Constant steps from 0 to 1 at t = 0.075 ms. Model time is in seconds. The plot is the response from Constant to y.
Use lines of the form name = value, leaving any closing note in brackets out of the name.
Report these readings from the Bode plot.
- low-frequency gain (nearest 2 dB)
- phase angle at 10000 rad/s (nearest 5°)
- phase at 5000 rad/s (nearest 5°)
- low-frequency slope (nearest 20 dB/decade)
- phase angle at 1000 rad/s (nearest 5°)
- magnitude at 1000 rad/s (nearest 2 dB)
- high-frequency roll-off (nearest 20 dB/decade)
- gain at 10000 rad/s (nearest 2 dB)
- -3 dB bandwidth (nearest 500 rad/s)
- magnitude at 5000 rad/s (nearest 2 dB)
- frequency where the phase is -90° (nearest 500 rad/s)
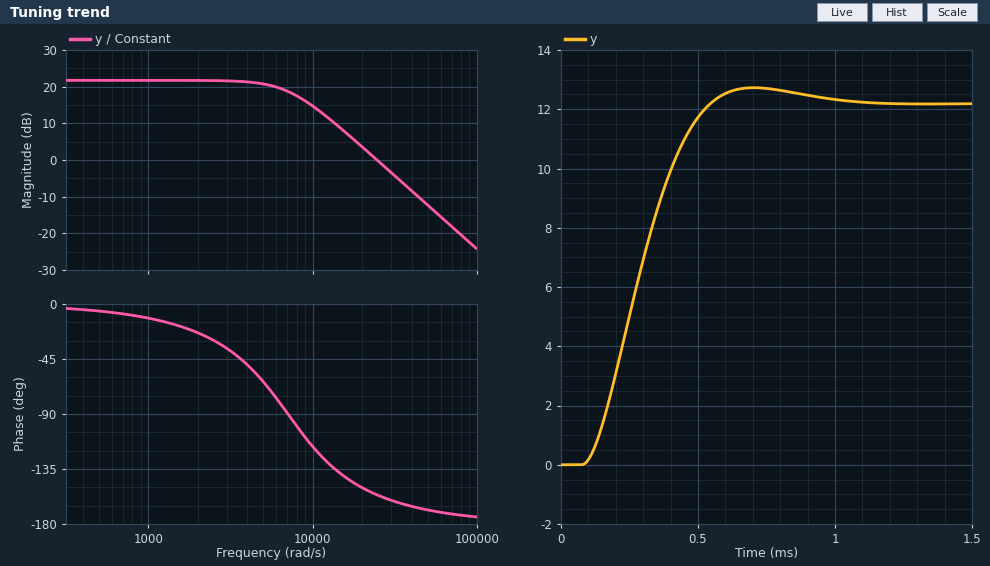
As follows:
low-frequency gain = 22 dB
phase angle at 10000 rad/s = -115°
phase at 5000 rad/s = -65°
low-frequency slope = 0 dB/decade
phase angle at 1000 rad/s = -10°
magnitude at 1000 rad/s = 22 dB
high-frequency roll-off = -40 dB/decade
gain at 10000 rad/s = 14 dB
-3 dB bandwidth = 7000 rad/s
magnitude at 5000 rad/s = 20 dB
frequency where the phase is -90° = 7000 rad/s
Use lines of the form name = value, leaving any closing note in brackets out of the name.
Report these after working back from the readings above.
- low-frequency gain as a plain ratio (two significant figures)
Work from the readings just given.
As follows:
low-frequency gain as a plain ratio = 13
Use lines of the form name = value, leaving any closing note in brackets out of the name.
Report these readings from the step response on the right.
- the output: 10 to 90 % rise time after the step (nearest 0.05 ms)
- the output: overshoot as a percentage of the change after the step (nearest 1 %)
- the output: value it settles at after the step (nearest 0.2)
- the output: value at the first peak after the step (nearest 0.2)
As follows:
the output: 10 to 90 % rise time after the step = 0.30 ms
the output: overshoot as a percentage of the change after the step = 4 %
the output: value it settles at after the step = 12.2
the output: value at the first peak after the step = 12.8
